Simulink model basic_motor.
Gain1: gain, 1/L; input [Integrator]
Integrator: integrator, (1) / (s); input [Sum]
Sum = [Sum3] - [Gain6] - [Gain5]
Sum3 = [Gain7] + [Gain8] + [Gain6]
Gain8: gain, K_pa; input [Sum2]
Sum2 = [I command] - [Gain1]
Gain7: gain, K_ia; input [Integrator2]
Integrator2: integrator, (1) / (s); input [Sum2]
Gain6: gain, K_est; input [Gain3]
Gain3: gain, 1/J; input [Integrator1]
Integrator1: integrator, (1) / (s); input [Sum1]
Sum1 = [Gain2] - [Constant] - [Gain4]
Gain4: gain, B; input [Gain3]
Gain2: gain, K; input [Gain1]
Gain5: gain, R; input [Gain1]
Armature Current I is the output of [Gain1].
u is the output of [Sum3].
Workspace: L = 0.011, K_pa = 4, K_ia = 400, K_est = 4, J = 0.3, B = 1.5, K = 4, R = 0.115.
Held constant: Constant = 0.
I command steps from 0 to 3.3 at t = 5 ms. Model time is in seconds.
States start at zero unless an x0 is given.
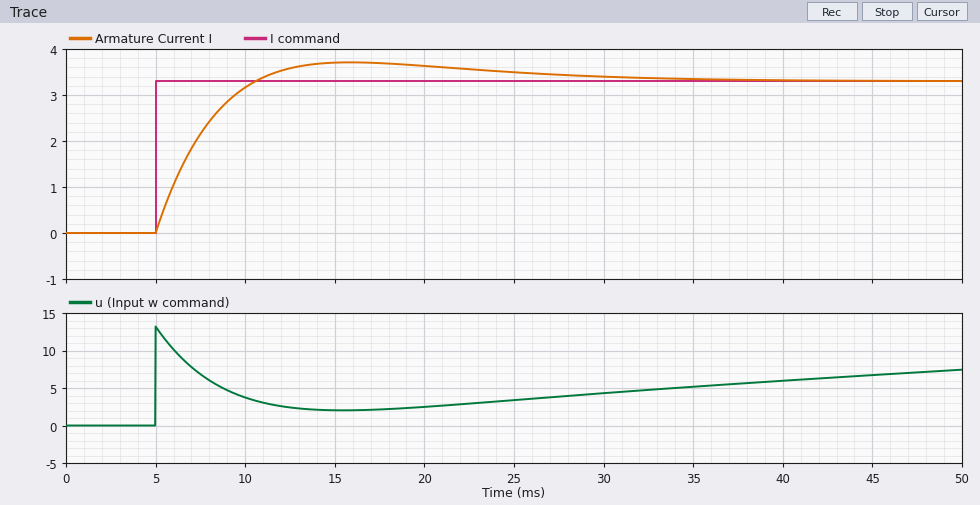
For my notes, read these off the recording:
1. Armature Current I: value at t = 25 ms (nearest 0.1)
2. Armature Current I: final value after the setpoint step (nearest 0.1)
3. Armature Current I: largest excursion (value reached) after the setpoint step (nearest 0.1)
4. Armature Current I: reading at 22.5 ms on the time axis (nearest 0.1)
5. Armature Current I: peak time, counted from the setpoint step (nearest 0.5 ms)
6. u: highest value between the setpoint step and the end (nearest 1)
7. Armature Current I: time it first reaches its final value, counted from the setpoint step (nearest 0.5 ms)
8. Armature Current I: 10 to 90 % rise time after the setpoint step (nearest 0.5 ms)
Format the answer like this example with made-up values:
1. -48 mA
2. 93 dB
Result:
1. 3.5
2. 3.3
3. 3.7
4. 3.6
5. 11.0 ms
6. 13
7. 5.5 ms
8. 4.0 ms
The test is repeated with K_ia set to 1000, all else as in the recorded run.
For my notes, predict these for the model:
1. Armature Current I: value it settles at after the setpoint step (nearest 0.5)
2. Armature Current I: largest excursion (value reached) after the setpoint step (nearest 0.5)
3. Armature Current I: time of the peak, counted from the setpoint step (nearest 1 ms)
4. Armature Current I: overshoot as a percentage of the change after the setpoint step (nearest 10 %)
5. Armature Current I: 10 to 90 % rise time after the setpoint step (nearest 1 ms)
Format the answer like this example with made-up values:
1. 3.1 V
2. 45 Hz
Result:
1. 3.5
2. 4.0
3. 8 ms
4. 20 %
5. 3 ms
